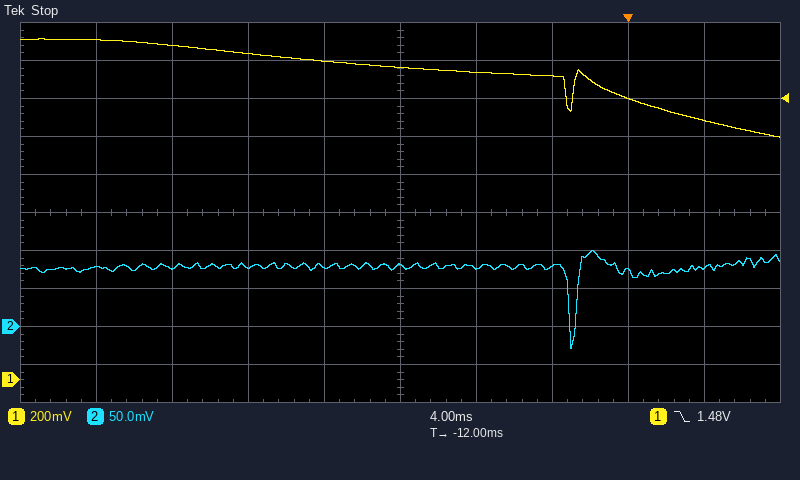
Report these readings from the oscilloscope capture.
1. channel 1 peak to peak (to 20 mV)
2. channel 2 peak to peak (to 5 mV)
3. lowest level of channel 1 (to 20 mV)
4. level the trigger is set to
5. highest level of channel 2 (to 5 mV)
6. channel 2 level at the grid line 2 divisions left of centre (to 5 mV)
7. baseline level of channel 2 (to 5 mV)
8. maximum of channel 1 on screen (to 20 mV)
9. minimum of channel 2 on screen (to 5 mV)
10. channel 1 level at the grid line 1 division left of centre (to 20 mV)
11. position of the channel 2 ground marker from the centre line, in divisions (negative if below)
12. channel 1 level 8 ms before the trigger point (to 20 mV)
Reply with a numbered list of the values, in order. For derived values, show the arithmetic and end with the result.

1. 1.80 V − (1.28 V) = 520 mV
2. 100 mV − (-30 mV) = 130 mV
3. 1.28 V
4. 1.48 V
5. 100 mV
6. 80 mV
7. 80 mV
8. 1.80 V
9. -30 mV
10. 1.68 V
11. -3.0 div
12. 1.62 V
